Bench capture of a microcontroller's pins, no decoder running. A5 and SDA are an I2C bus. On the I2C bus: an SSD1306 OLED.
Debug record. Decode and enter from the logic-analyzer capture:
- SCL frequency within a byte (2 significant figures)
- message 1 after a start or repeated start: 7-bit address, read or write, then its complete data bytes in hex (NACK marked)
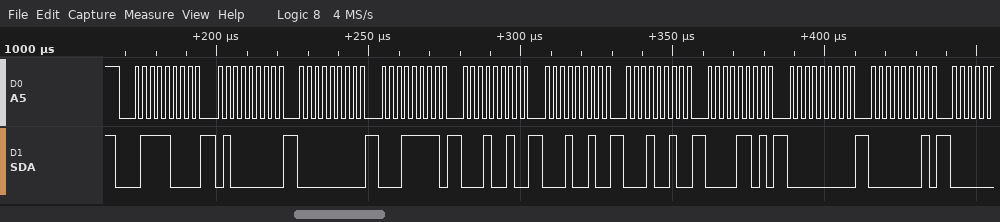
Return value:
400 kHz
0x3C write: 40 00 1F 12 12 12 0D 00 01
